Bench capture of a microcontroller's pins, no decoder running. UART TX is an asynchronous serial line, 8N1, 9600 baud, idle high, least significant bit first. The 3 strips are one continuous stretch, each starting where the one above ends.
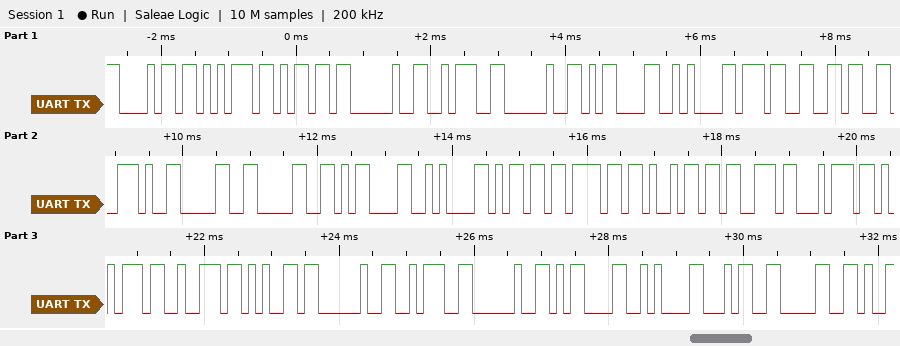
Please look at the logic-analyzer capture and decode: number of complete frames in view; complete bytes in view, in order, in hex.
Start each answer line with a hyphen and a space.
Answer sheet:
- 30
- 68 75 6D 20 3A 20 0D 0A 37 36 2E 30 30 0D 0A 6D 6F 69 73 74 75 72 65 20 3A 20 0D 0A 34 30
